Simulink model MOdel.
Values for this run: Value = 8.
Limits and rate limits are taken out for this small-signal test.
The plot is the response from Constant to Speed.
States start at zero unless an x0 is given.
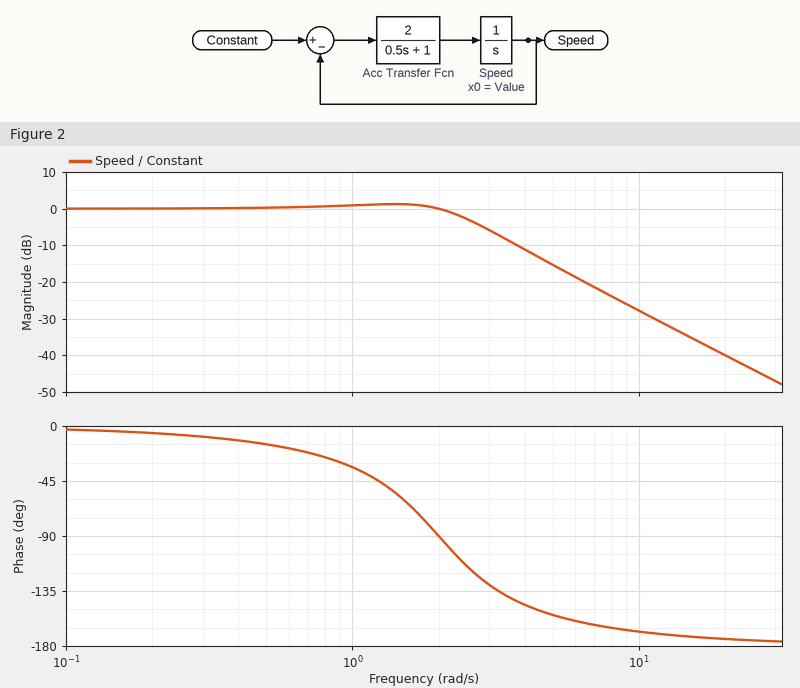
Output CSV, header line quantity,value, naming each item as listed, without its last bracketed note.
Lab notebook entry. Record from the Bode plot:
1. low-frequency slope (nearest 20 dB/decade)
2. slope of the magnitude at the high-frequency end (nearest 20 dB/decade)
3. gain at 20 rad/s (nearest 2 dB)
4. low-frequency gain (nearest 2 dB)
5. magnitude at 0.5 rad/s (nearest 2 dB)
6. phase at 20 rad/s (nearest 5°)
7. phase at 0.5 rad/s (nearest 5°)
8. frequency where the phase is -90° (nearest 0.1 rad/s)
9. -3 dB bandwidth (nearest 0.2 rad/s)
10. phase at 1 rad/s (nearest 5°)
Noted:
quantity,value
low-frequency slope,0 dB/decade
slope of the magnitude at the high-frequency end,-40 dB/decade
gain at 20 rad/s,-40 dB
low-frequency gain,0 dB
magnitude at 0.5 rad/s,0 dB
phase at 20 rad/s,-175°
phase at 0.5 rad/s,-15°
frequency where the phase is -90°,2.0 rad/s
-3 dB bandwidth,2.6 rad/s
phase at 1 rad/s,-35°
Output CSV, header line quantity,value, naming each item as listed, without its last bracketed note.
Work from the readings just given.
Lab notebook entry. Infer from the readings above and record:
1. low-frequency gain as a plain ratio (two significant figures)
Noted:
quantity,value
low-frequency gain as a plain ratio,1.0
